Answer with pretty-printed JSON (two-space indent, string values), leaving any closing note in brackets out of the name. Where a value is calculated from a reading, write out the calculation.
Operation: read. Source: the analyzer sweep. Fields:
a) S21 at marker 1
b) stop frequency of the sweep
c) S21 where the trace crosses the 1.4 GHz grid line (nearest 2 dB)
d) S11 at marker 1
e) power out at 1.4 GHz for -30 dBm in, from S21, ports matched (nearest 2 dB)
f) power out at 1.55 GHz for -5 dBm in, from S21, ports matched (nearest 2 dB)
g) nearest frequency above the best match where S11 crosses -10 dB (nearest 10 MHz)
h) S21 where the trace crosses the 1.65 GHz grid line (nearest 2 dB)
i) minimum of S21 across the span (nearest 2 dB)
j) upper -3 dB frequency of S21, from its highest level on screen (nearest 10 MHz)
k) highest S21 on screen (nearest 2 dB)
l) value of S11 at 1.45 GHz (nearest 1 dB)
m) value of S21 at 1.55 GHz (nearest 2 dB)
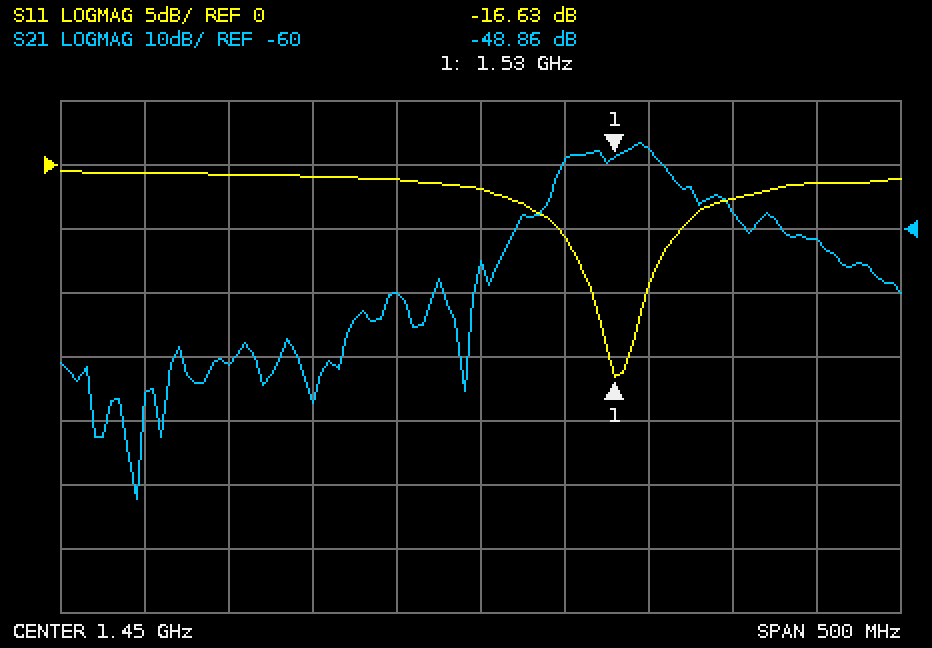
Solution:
{
  "S21 at marker 1": "-48.86 dB",
  "stop frequency of the sweep": "1.7 GHz",
  "S21 where the trace crosses the 1.4 GHz grid line": "-70 dB",
  "S11 at marker 1": "-16.63 dB",
  "power out at 1.4 GHz for -30 dBm in, from S21, ports matched": "-30 dBm + (-70 dB) = -100 dBm",
  "power out at 1.55 GHz for -5 dBm in, from S21, ports matched": "-5 dBm + (-48 dB) = -52 dBm",
  "nearest frequency above the best match where S11 crosses -10 dB": "1.55 GHz",
  "S21 where the trace crosses the 1.65 GHz grid line": "-62 dB",
  "minimum of S21 across the span": "-102 dB",
  "upper -3 dB frequency of S21, from its highest level on screen": "1.56 GHz",
  "highest S21 on screen": "-46 dB",
  "value of S11 at 1.45 GHz": "-2 dB",
  "value of S21 at 1.55 GHz": "-48 dB"
}
